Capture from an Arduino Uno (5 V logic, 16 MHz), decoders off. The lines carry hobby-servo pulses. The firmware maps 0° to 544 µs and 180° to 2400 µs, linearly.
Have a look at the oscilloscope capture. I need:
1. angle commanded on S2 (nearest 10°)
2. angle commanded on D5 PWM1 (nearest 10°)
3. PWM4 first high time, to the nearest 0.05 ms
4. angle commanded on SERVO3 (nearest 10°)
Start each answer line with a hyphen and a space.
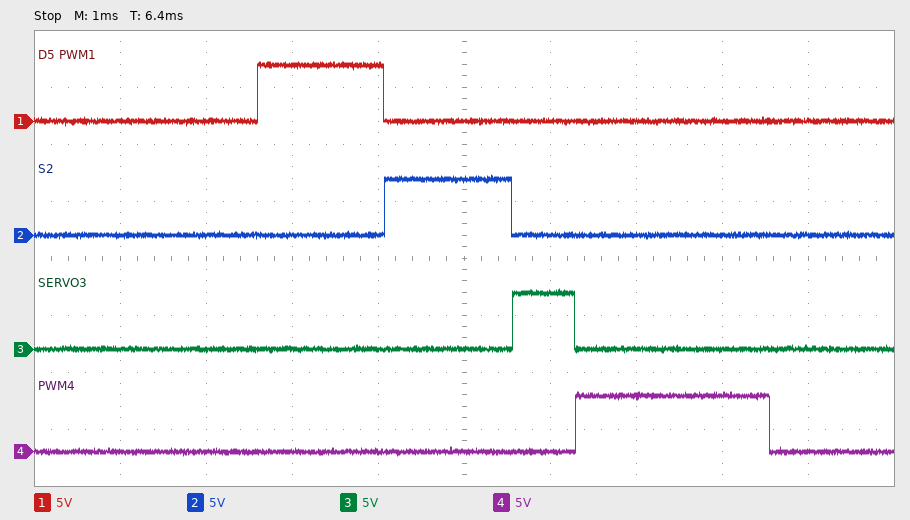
- 90°
- 90°
- 2.25 ms
- 20°
